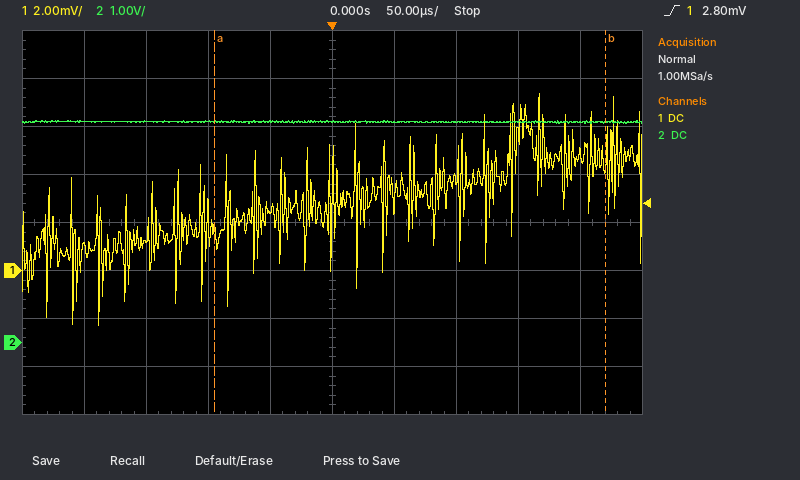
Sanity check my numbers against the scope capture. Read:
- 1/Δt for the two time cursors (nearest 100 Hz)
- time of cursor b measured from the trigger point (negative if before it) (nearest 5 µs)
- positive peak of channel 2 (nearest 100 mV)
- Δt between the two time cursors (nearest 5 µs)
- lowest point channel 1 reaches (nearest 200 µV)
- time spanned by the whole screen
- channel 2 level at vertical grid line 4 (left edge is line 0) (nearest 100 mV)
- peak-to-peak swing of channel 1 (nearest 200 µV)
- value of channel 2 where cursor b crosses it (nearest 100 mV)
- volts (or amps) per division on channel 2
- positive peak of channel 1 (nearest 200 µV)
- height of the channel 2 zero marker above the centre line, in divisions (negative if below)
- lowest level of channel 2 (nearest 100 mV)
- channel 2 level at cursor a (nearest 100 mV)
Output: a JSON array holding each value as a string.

["3.2 kHz", "+220 µs", "4.6 V", "315 µs", "-2.2 mV", "500 µs", "4.6 V", "9.6 mV", "4.6 V", "1 V", "7.4 mV", "-2.5 div", "4.6 V", "4.6 V"]
